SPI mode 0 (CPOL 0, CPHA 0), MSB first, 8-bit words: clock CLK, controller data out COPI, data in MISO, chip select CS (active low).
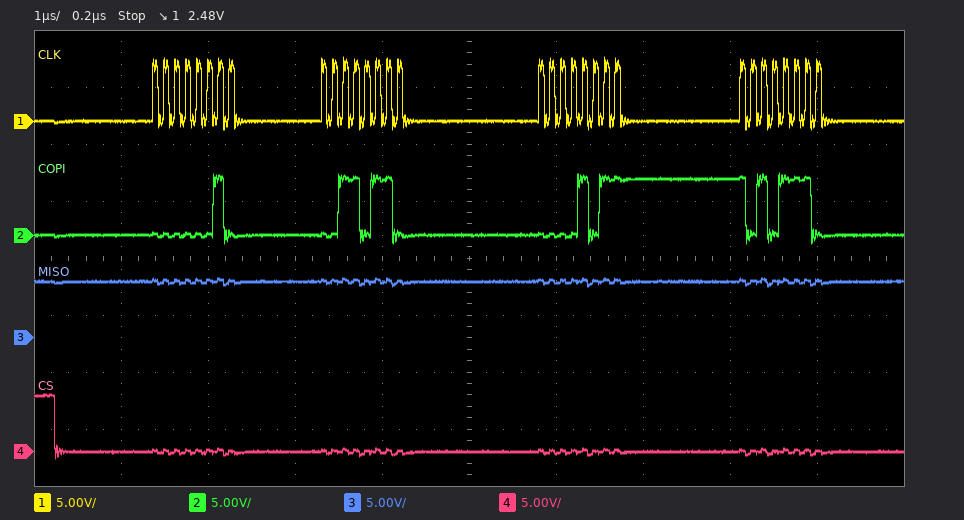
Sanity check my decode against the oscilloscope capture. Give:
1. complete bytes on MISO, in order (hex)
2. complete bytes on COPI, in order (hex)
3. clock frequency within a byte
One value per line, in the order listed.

FF FF FF FF
02 36 0B AE
8 MHz
